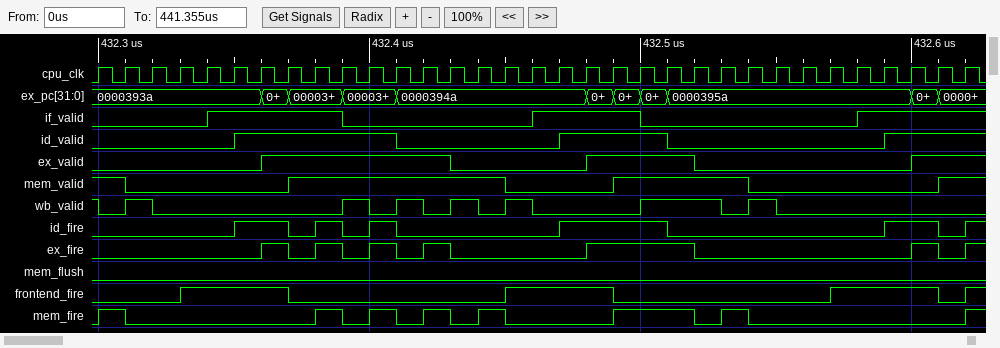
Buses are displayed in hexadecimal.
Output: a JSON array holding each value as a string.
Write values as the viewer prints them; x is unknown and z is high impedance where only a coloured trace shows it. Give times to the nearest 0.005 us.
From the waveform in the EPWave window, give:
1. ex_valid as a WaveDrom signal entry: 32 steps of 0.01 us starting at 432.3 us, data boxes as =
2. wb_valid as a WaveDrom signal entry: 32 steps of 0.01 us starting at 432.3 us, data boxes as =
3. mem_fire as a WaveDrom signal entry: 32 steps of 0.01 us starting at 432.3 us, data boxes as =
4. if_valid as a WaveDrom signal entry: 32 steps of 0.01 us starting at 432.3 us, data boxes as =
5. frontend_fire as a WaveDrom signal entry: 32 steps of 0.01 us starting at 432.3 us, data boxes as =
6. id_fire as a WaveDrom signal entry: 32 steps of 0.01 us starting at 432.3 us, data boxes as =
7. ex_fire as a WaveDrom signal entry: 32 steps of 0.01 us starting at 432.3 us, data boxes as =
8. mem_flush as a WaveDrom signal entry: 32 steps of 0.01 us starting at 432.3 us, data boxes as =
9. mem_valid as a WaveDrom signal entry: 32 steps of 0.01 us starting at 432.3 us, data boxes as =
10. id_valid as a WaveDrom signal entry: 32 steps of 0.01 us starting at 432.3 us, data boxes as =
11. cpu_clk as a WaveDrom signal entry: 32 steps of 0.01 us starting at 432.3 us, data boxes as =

["{name: 'ex_valid', wave: '0.....1......0....1...0.......1.'}", "{name: 'wb_valid', wave: '010......10101010...1..010......'}", "{name: 'mem_fire', wave: '10......10101010...1..010.......'}", "{name: 'if_valid', wave: '0...1....0......1...0.......1...'}", "{name: 'frontend_fire', wave: '0..1...0.......1...0.......1...0'}", "{name: 'id_fire', wave: '0....1.01010.....1...0.......1.0'}", "{name: 'ex_fire', wave: '0.....10101010....1...0.......10'}", "{name: 'mem_flush', wave: '0...............................'}", "{name: 'mem_valid', wave: '10.....1.......0...1....0......1'}", "{name: 'id_valid', wave: '0....1.....0.....1...0.......1..'}", "{name: 'cpu_clk', wave: 'p...............................'}"]
